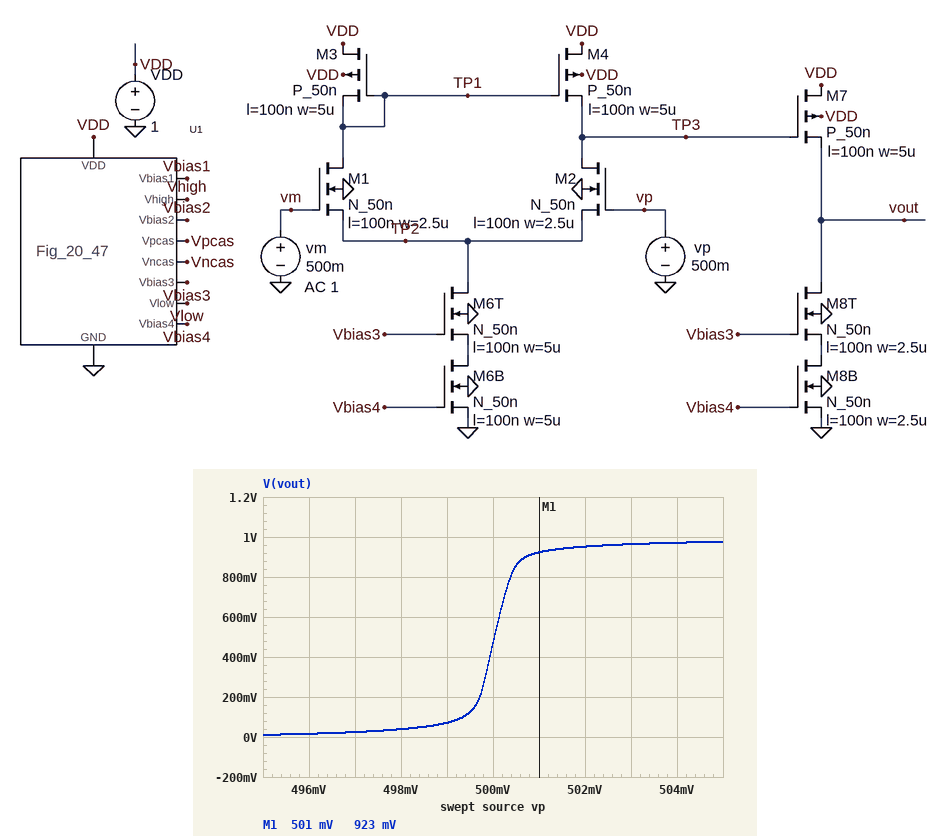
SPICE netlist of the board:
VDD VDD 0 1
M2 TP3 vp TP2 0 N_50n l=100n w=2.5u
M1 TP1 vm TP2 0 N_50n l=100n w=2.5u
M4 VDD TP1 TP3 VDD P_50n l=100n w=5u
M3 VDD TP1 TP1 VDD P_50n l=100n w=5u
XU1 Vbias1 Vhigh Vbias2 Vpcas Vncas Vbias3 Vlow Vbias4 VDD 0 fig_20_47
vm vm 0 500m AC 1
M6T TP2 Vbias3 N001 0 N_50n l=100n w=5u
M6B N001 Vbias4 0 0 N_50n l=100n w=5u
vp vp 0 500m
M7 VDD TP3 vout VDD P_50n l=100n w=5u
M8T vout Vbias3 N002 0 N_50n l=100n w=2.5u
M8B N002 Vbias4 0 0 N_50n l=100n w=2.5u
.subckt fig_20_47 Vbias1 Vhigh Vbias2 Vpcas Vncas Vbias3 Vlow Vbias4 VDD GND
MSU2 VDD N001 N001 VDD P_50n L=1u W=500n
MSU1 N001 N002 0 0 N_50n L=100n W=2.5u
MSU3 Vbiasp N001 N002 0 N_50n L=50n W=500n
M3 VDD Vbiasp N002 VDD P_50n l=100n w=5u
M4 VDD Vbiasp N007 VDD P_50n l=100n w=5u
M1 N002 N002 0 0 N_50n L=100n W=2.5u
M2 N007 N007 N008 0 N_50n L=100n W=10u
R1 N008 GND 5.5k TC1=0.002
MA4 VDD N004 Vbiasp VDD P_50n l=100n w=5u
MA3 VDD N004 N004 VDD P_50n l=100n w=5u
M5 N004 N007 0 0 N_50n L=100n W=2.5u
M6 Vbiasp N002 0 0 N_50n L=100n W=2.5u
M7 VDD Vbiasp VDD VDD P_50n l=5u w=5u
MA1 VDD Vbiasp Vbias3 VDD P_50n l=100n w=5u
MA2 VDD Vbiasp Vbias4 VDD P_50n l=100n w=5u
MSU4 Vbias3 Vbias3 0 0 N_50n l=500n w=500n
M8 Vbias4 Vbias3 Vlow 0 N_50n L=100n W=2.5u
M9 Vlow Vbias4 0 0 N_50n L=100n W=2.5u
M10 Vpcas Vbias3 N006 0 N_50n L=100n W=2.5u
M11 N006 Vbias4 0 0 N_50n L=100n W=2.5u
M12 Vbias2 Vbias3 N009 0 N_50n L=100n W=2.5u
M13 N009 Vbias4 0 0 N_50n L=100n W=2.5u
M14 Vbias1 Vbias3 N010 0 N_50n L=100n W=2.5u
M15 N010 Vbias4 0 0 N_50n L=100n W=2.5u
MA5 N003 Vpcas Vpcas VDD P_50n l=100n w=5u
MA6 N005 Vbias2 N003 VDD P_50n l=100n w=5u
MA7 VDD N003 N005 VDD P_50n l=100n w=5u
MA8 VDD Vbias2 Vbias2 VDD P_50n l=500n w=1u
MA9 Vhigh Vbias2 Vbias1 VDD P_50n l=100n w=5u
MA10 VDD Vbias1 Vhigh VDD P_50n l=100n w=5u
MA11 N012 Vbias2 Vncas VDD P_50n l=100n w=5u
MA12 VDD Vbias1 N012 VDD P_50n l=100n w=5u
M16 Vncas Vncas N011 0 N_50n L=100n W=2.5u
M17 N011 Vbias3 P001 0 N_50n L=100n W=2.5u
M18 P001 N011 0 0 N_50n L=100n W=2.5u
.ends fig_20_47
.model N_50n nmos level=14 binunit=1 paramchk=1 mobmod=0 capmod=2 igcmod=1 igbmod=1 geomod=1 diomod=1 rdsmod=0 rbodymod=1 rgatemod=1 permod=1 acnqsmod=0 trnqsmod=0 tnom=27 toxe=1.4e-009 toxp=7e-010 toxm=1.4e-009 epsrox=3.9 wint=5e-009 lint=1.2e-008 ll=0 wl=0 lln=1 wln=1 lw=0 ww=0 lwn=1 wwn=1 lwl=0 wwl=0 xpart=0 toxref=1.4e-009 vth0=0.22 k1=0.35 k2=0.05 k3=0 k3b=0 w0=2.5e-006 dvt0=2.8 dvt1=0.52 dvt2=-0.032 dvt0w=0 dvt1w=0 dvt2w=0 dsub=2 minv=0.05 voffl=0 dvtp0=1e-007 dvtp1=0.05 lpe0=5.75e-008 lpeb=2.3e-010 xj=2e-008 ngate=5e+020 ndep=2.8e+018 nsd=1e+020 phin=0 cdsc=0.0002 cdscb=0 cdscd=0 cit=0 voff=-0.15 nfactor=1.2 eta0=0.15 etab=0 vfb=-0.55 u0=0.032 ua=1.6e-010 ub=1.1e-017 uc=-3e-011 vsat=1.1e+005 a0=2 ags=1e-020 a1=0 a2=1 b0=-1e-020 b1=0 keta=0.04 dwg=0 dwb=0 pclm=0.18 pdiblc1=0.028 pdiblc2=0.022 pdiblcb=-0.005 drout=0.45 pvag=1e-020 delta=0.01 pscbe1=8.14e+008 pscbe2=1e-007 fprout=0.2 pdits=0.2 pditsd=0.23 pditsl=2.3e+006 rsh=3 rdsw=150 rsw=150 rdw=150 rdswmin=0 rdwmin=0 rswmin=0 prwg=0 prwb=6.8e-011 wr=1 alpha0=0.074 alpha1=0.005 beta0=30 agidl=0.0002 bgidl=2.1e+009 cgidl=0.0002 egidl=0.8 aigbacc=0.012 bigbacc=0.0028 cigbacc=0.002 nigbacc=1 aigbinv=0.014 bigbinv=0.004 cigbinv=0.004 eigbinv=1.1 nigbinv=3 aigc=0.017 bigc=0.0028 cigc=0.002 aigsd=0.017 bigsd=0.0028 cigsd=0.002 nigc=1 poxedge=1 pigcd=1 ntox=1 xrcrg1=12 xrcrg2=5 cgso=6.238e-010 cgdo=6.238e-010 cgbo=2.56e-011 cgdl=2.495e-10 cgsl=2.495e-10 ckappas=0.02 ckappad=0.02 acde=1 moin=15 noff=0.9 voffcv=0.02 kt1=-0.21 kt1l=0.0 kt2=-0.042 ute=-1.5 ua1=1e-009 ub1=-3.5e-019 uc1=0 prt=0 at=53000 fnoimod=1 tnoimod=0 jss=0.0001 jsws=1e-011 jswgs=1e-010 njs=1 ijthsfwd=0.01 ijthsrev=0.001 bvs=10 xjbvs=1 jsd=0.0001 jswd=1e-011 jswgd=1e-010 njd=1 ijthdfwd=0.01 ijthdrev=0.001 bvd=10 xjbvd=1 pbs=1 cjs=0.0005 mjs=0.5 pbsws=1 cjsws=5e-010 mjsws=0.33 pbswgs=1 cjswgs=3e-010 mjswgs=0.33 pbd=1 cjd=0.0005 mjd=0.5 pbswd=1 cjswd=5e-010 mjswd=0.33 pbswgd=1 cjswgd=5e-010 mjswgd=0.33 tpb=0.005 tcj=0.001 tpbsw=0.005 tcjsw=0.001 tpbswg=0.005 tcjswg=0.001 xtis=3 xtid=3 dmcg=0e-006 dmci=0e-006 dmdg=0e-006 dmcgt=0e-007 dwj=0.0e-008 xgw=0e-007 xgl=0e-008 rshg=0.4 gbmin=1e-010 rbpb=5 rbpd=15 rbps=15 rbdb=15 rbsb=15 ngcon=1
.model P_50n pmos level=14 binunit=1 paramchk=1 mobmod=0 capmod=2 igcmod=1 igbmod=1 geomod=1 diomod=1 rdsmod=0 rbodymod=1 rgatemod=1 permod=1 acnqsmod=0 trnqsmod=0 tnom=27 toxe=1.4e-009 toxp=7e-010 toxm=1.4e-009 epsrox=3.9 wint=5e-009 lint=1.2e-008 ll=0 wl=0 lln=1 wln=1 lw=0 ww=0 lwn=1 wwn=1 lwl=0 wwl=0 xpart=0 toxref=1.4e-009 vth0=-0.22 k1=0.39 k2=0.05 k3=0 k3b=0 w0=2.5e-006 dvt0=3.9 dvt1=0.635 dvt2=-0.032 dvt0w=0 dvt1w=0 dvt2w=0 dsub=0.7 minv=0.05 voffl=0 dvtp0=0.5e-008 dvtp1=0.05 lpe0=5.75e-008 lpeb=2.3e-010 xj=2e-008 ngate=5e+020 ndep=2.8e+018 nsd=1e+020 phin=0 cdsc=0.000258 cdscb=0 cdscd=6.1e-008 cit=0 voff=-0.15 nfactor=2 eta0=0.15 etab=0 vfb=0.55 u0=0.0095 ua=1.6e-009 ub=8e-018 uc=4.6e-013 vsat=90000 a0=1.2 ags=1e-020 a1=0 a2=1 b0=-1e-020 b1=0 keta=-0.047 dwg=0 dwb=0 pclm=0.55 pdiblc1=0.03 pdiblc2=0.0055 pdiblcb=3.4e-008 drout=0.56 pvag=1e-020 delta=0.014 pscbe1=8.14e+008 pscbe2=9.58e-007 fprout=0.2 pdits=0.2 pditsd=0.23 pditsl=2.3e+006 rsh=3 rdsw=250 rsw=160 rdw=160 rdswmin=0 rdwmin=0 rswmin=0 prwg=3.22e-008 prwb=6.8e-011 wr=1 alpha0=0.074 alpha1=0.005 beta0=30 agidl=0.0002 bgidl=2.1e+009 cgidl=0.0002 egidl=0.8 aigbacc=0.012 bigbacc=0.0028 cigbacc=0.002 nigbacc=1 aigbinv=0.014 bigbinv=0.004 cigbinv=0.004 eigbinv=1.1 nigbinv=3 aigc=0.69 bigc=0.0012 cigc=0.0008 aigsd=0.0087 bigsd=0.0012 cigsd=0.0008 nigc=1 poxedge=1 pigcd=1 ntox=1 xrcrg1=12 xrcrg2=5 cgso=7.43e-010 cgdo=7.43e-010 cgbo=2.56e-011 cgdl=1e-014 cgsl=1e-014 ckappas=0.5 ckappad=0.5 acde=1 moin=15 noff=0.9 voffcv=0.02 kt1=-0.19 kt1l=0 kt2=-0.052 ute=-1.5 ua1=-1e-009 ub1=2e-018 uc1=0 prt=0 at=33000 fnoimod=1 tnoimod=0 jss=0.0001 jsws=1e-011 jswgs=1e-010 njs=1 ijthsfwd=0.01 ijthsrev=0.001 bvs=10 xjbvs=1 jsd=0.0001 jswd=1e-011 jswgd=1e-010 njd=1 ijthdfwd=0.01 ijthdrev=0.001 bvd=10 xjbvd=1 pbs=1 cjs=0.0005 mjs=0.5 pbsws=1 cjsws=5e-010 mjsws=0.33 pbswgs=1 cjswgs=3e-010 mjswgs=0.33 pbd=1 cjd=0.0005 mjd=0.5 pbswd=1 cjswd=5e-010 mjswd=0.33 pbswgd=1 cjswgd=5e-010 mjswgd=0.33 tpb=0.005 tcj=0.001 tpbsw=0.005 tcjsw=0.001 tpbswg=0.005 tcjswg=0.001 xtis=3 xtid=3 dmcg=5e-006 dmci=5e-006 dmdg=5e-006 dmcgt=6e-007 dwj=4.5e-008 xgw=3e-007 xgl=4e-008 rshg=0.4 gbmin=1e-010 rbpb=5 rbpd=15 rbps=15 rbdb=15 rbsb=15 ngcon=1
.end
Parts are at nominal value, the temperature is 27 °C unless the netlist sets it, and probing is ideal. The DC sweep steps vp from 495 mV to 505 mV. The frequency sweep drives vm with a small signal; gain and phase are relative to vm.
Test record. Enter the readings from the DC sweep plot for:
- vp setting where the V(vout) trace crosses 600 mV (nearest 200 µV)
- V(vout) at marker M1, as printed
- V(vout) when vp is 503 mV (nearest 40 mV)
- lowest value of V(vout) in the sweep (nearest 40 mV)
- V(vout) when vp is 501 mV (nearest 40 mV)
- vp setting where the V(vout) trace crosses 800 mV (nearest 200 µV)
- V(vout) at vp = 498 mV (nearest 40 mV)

500.2 mV
923 mV
960 mV
0 V
920 mV
500.4 mV
40 mV
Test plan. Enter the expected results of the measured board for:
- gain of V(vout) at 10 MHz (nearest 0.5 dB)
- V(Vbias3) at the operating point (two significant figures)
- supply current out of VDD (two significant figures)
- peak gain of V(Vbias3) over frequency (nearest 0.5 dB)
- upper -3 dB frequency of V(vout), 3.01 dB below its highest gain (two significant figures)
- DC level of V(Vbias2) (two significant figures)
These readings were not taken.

51.0 dB
540 mV
140 µA
1.0 dB
3.7 MHz
370 mV
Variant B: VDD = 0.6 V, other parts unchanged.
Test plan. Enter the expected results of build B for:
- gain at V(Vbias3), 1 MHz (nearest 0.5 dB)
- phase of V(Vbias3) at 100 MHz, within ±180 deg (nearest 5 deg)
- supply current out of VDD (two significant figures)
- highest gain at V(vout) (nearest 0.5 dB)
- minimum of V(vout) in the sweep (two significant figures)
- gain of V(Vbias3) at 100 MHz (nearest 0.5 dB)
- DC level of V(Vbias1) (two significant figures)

-22.0 dB
90 deg
110 µA
47.0 dB
14 mV
-5.5 dB
240 mV
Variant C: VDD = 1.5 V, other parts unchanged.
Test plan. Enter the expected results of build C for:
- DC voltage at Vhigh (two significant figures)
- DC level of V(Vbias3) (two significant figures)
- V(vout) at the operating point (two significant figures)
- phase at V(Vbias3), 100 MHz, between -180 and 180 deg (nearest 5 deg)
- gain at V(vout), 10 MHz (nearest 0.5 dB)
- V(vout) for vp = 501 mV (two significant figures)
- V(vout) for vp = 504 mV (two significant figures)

1.3 V
550 mV
970 mV
80 deg
51.5 dB
1.4 V
1.5 V
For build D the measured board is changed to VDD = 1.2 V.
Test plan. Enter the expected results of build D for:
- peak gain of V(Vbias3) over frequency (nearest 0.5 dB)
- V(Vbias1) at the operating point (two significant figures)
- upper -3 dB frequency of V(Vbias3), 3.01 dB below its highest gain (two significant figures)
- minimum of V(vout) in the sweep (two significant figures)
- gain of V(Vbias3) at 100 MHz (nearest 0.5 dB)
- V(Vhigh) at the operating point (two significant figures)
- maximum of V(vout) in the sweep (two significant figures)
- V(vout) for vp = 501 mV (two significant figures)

0.5 dB
840 mV
66 MHz
12 mV
-5.0 dB
980 mV
1.2 V
1.1 V
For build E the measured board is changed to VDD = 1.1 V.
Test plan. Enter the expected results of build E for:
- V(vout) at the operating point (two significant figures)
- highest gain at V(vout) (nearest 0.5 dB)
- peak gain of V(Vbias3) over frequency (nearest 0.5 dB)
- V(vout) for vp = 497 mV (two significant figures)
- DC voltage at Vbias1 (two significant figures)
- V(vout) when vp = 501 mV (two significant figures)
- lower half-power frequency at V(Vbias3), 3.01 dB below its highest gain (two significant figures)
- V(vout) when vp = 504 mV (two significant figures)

570 mV
60.5 dB
1.0 dB
26 mV
740 mV
1.0 V
3.3 MHz
1.1 V
